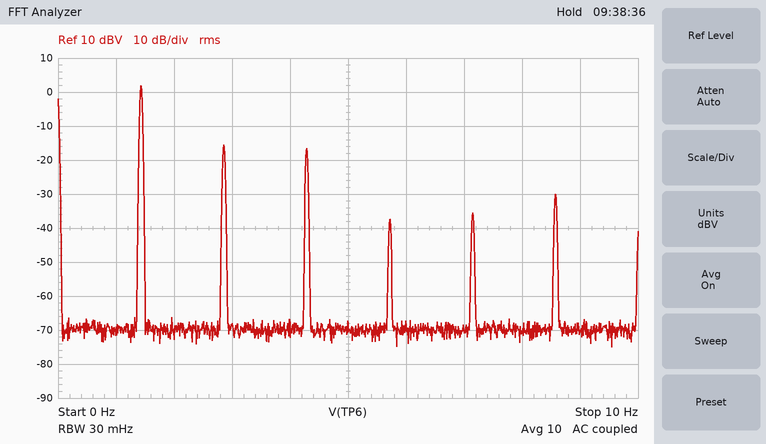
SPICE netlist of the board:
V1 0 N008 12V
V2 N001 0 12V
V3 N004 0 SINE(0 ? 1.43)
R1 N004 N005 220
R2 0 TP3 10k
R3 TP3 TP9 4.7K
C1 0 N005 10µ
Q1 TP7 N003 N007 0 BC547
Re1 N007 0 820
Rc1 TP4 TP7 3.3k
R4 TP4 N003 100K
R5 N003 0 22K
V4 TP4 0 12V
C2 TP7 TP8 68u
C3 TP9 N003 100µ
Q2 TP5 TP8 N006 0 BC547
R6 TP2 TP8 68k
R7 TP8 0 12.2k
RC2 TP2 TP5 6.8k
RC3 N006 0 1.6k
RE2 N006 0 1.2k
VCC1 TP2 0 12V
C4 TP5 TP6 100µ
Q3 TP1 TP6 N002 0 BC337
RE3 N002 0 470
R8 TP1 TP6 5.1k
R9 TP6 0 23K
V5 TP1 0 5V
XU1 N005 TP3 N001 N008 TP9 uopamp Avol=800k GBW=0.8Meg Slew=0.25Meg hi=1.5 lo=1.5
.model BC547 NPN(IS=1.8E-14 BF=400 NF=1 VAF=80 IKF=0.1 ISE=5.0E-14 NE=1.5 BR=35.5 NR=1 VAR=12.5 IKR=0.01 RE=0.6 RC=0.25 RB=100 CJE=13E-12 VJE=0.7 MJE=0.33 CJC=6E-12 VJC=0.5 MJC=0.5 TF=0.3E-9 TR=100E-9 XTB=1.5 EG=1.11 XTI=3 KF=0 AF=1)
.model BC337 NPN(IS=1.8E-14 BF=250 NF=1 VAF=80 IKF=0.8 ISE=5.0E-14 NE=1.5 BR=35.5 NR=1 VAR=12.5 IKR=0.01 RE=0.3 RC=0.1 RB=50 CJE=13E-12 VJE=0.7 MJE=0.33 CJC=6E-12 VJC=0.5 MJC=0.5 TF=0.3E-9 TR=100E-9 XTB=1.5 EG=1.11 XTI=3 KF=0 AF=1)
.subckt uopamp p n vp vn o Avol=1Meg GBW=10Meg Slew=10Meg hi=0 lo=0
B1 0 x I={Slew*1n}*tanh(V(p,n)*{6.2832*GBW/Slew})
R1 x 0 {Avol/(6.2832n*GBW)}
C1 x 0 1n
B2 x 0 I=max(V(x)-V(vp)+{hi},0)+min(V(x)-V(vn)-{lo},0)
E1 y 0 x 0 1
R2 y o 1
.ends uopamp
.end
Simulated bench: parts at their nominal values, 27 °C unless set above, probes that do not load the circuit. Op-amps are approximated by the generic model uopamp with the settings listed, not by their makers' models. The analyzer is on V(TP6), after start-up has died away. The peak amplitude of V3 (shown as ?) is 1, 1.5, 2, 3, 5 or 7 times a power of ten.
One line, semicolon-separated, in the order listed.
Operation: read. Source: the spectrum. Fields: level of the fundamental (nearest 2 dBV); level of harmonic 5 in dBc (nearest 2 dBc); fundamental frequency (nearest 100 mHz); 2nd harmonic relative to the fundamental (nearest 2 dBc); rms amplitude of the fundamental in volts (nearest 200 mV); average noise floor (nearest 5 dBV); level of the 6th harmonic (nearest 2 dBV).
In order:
2 dBV; -38 dBc; 1.4 Hz; -18 dBc; 1.2 V; -70 dBV; -30 dBV
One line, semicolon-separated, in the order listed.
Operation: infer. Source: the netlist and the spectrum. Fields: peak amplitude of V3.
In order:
150 mV
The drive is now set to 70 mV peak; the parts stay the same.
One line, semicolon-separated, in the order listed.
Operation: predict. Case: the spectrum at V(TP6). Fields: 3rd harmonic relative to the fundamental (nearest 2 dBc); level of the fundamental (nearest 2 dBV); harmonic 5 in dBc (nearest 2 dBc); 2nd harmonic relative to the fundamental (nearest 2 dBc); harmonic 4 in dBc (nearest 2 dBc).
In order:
-22 dBc; -4 dBV; -36 dBc; -16 dBc; -34 dBc
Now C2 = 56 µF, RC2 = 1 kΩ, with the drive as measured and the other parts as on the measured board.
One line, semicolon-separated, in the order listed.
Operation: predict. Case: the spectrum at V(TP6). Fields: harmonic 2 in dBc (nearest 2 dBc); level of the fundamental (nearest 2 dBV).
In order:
-50 dBc; -6 dBV
